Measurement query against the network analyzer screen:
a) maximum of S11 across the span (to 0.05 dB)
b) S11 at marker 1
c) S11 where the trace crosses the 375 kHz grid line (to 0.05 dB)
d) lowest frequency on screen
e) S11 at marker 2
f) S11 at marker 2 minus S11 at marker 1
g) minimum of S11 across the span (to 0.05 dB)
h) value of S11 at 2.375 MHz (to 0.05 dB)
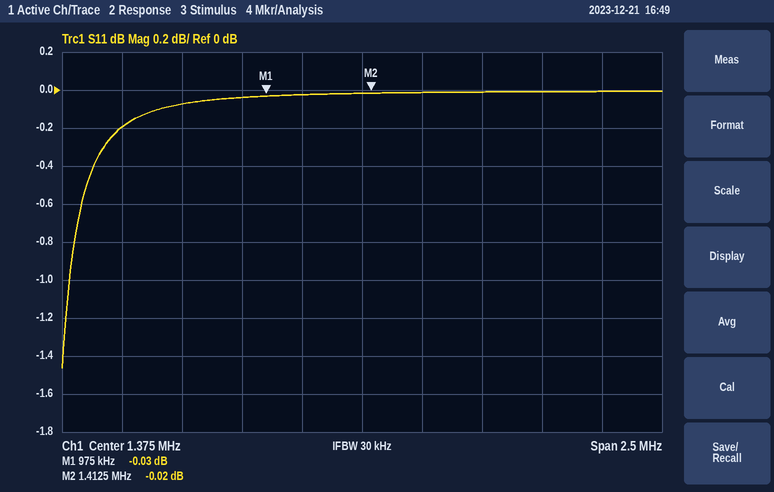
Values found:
0.00 dB
-0.03 dB
-0.20 dB
125 kHz
-0.02 dB
0.01 dB
-1.45 dB
0.00 dB
